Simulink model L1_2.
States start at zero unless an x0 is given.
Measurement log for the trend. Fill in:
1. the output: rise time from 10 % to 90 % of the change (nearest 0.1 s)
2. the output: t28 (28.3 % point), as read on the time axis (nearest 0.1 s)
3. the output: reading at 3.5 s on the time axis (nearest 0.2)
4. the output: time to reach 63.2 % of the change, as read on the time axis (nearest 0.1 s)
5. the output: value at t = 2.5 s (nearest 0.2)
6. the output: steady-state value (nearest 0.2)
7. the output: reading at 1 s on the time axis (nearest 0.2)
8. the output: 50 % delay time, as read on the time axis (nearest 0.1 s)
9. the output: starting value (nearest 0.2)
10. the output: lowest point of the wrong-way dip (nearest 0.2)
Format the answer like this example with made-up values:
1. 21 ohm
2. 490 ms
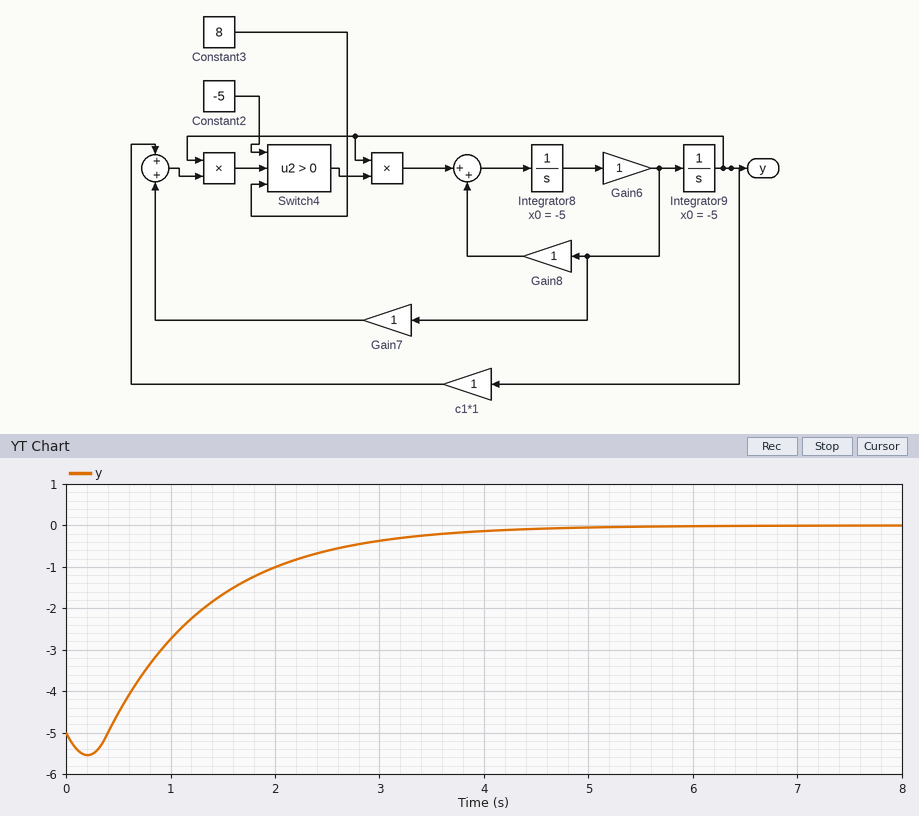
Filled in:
1. 2.2 s
2. 0.7 s
3. -0.2
4. 1.4 s
5. -0.6
6. 0.0
7. -2.8
8. 1.1 s
9. -5.0
10. -5.6
